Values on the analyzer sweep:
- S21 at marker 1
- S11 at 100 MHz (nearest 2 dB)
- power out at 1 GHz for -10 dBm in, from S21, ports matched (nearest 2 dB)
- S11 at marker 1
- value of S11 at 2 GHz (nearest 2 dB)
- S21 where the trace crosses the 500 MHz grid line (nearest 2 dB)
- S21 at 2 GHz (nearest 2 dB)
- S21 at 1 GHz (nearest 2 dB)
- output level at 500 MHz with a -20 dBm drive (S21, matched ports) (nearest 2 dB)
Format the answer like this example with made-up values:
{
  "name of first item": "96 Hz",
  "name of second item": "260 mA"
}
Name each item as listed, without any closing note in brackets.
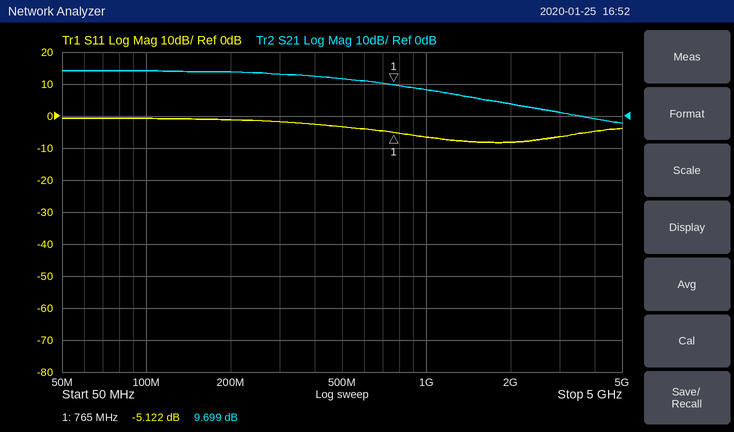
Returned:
{
  "S21 at marker 1": "9.699 dB",
  "S11 at 100 MHz": "0 dB",
  "power out at 1 GHz for -10 dBm in, from S21, ports matched": "-2 dBm",
  "S11 at marker 1": "-5.122 dB",
  "value of S11 at 2 GHz": "-8 dB",
  "S21 where the trace crosses the 500 MHz grid line": "12 dB",
  "S21 at 2 GHz": "4 dB",
  "S21 at 1 GHz": "8 dB",
  "output level at 500 MHz with a -20 dBm drive (S21, matched ports)": "-8 dBm"
}
